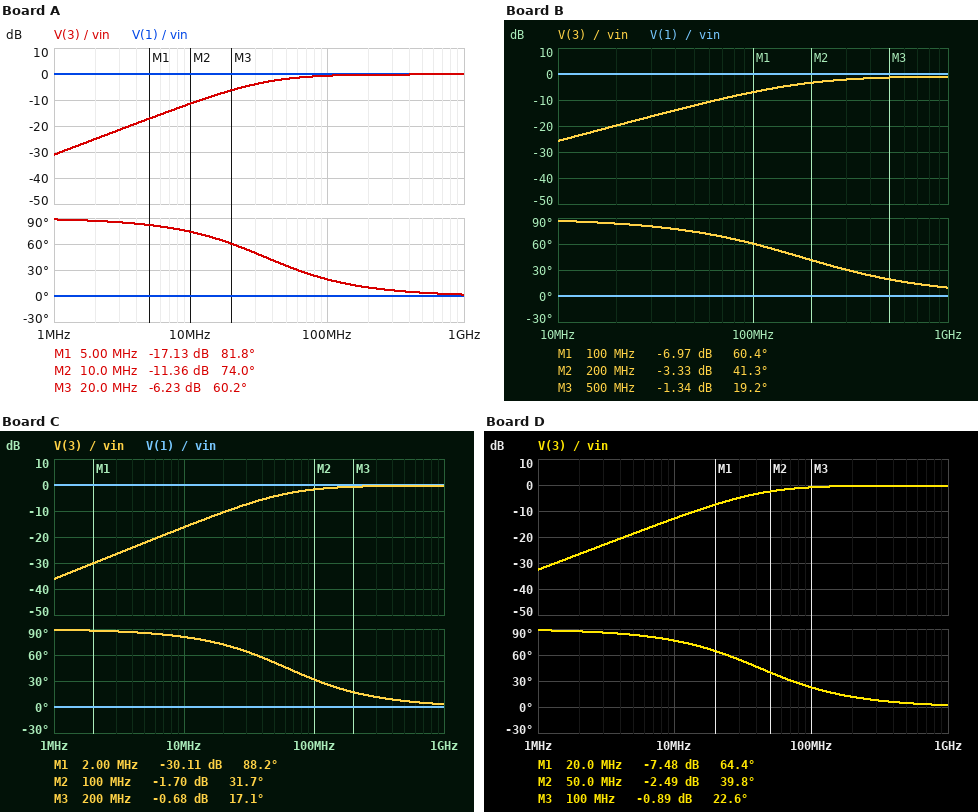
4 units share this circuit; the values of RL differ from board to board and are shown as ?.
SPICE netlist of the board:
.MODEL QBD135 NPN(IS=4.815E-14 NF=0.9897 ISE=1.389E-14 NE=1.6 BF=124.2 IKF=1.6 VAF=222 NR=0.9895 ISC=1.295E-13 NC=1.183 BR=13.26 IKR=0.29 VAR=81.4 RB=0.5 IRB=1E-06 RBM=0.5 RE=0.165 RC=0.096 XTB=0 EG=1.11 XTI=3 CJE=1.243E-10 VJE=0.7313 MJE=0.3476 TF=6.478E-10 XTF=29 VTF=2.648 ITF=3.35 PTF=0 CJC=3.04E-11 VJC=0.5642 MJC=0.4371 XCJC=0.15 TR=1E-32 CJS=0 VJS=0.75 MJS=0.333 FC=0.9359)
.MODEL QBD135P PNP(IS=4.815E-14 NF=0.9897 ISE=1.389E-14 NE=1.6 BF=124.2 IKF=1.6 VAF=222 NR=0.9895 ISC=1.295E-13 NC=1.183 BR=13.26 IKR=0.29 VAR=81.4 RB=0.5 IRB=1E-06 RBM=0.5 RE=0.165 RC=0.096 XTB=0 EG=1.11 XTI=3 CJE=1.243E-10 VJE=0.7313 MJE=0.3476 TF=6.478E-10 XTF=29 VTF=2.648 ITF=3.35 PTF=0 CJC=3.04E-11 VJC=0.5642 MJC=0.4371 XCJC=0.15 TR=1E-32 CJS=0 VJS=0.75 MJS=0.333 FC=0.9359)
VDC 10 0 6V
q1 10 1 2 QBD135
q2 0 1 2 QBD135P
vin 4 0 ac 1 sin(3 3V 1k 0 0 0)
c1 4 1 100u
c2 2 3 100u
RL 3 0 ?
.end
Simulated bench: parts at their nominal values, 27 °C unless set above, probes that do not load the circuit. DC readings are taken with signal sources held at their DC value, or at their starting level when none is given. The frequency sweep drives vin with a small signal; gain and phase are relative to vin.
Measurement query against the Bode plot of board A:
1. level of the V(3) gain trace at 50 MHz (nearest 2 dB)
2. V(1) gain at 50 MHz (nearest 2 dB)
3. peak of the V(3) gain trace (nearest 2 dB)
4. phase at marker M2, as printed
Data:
-2 dB
0 dB
0 dB
74.0 deg
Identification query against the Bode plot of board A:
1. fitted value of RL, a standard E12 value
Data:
18 Ω
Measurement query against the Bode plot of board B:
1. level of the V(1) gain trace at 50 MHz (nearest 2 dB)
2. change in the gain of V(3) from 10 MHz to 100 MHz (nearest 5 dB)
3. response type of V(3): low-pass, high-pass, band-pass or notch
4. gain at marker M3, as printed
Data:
0 dB
20 dB
high-pass
-1.34 dB
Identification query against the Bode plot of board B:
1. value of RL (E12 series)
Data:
3.3 Ω
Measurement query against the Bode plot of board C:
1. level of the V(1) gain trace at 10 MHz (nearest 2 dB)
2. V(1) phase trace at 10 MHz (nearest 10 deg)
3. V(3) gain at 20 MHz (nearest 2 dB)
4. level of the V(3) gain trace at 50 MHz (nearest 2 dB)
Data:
0 dB
0 deg
-10 dB
-4 dB
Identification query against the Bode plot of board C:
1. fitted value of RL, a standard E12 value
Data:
10 Ω
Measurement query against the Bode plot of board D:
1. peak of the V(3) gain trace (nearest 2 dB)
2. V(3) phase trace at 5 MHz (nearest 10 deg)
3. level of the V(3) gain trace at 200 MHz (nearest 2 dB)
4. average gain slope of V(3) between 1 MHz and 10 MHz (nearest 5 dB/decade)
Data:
0 dB
80 deg
0 dB
20 dB/decade
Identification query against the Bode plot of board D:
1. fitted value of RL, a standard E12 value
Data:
15 Ω
